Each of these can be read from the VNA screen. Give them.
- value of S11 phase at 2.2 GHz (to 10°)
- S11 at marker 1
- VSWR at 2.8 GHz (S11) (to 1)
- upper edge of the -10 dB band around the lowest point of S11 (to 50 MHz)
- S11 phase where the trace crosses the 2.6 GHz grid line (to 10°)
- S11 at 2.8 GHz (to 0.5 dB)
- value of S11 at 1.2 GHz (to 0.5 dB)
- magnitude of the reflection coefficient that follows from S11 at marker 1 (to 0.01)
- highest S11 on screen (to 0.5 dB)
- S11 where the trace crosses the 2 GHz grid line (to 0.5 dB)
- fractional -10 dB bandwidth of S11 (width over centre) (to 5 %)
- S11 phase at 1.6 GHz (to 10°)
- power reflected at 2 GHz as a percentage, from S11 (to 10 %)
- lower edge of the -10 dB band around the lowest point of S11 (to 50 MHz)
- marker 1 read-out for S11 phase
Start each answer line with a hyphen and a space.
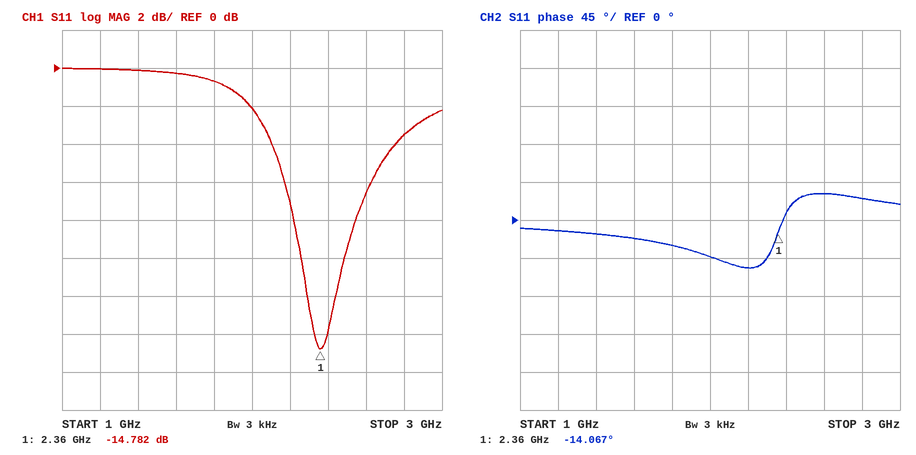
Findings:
- -60°
- -14.782 dB
- 5
- 2.50 GHz
- 30°
- -3.5 dB
- 0.0 dB
- 0.18
- 0.0 dB
- -2.0 dB
- 10 %
- -20°
- 60 %
- 2.25 GHz
- -14.067°
